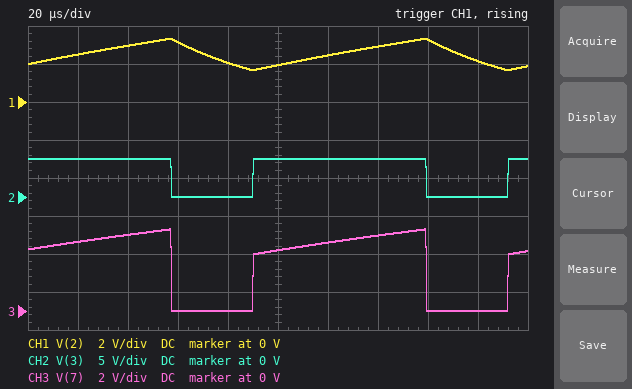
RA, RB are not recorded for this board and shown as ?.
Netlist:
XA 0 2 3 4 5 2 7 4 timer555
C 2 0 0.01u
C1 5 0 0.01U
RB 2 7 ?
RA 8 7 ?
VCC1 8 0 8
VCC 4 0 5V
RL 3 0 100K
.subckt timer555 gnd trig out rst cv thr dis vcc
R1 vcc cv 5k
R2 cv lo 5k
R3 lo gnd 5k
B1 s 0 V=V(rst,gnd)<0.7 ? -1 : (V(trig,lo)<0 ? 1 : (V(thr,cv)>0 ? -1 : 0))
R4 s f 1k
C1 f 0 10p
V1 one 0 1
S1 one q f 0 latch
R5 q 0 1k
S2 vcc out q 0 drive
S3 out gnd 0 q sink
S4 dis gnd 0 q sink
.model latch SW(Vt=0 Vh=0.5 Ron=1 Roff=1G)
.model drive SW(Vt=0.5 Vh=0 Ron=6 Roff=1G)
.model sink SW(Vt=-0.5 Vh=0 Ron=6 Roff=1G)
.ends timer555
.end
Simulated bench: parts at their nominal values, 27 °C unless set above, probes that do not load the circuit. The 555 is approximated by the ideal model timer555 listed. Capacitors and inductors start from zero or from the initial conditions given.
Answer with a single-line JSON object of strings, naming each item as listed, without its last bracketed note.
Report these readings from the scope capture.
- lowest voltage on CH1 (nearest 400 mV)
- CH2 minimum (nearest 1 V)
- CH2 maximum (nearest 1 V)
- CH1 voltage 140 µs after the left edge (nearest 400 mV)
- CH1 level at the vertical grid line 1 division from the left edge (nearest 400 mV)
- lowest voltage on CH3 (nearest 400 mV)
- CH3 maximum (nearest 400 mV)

{"lowest voltage on CH1": "1.6 V", "CH2 minimum": "0 V", "CH2 maximum": "5 V", "CH1 voltage 140 µs after the left edge": "2.8 V", "CH1 level at the vertical grid line 1 division from the left edge": "2.4 V", "lowest voltage on CH3": "0 V", "CH3 maximum": "4.4 V"}
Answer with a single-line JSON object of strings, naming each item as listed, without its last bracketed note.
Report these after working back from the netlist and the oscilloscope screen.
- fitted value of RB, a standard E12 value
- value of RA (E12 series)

{"fitted value of RB, a standard E12 value": "4.7 kΩ", "value of RA": "18 kΩ"}
